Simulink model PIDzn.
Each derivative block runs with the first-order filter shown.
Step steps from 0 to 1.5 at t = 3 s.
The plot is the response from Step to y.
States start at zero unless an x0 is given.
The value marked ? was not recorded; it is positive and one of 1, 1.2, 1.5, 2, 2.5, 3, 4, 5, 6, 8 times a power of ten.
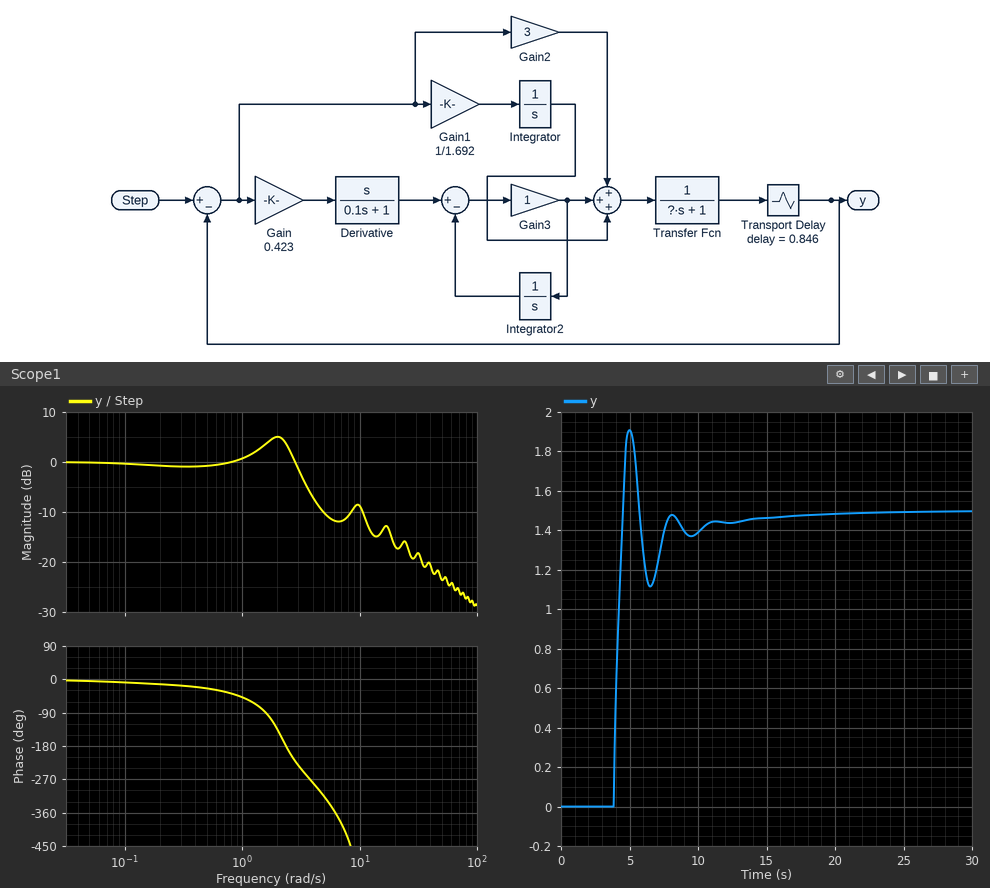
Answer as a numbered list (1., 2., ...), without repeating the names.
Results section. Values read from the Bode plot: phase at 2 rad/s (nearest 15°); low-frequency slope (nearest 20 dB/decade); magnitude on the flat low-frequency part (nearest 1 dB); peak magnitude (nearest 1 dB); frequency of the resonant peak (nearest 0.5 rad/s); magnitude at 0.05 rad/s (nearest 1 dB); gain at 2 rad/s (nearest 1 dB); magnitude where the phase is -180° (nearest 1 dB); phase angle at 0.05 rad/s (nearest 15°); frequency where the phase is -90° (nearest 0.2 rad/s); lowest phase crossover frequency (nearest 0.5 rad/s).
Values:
1. -135°
2. 0 dB/decade
3. 0 dB
4. 5 dB
5. 2.0 rad/s
6. 0 dB
7. 5 dB
8. 4 dB
9. 0°
10. 1.6 rad/s
11. 2.5 rad/s
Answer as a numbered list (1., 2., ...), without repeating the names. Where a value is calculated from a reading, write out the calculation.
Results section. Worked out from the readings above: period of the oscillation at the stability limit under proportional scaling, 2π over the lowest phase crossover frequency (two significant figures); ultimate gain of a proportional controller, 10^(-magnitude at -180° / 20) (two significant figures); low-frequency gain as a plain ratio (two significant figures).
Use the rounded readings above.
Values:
1. 2π / 2.5 = 2.5 s
2. 10^(-4 / 20) = 0.63
3. 10^(0 / 20) = 1.0
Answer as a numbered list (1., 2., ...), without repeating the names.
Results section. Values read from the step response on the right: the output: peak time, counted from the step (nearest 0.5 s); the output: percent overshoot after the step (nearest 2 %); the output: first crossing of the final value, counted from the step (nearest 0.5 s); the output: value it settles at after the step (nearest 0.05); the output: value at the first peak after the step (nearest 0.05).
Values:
1. 2.0 s
2. 28 %
3. 1.5 s
4. 1.50
5. 1.90
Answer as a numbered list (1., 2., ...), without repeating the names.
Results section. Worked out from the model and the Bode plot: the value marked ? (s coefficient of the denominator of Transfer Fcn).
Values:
1. 2
